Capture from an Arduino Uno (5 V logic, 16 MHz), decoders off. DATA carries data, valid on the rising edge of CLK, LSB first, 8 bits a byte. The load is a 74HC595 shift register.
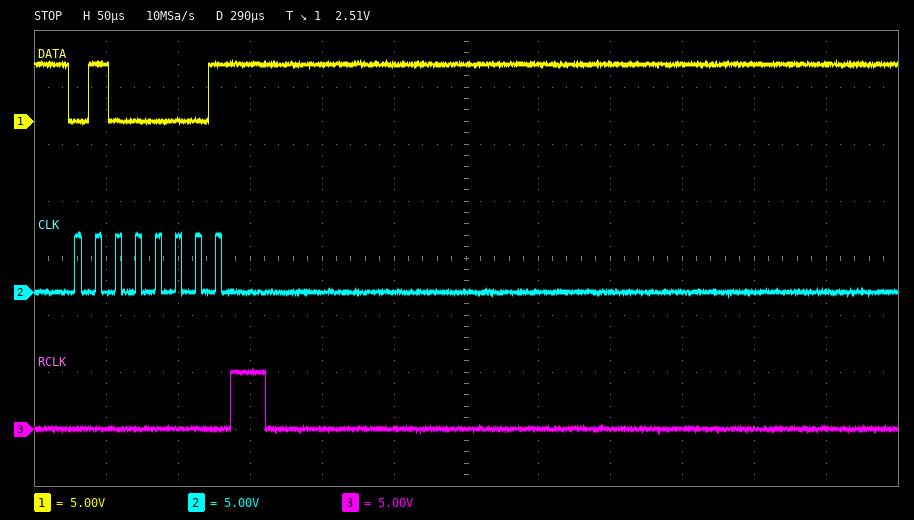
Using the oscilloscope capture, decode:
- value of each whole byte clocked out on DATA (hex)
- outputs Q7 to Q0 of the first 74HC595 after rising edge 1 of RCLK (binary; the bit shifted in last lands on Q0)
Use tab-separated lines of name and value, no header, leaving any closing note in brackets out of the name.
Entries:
value of each whole byte clocked out on DATA	82
outputs Q7 to Q0 of the first 74HC595 after rising edge 1 of RCLK	01000001
